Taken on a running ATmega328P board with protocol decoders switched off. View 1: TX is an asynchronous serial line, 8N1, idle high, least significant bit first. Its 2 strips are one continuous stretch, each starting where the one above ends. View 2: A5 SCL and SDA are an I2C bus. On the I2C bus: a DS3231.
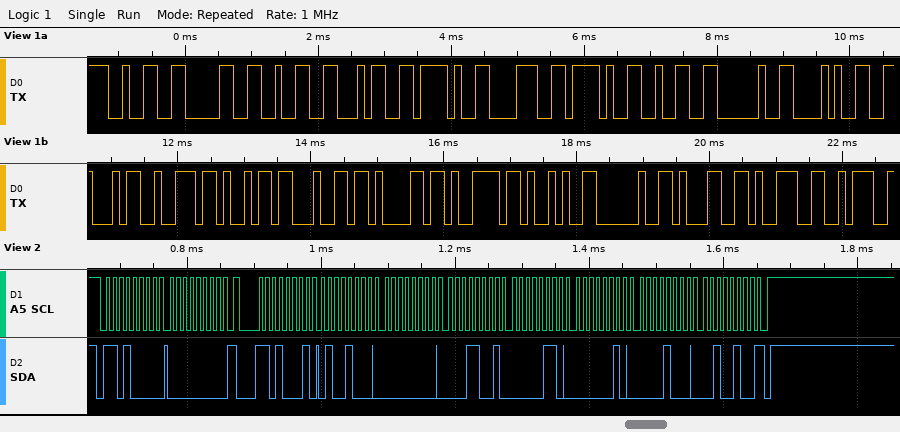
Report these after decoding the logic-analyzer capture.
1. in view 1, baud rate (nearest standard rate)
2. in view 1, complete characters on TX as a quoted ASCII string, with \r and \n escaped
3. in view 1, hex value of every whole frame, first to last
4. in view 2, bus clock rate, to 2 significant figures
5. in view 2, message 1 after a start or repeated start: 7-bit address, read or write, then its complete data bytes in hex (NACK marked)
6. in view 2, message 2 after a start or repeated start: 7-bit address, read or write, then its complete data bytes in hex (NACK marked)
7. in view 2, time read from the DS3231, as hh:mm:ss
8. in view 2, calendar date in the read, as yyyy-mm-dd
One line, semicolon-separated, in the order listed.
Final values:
9600 baud; "2024/8/2 (Friday) 19:"; 0x32 0x30 0x32 0x34 0x2F 0x38 0x2F 0x32 0x20 0x28 0x46 0x72 0x69 0x64 0x61 0x79 0x29 0x20 0x31 0x39 0x3A; 100 kHz; 0x68 write: 00; 0x68 read: 48 00 19 06 02 08 24 NACK; 19:00:48; 2024-08-02
